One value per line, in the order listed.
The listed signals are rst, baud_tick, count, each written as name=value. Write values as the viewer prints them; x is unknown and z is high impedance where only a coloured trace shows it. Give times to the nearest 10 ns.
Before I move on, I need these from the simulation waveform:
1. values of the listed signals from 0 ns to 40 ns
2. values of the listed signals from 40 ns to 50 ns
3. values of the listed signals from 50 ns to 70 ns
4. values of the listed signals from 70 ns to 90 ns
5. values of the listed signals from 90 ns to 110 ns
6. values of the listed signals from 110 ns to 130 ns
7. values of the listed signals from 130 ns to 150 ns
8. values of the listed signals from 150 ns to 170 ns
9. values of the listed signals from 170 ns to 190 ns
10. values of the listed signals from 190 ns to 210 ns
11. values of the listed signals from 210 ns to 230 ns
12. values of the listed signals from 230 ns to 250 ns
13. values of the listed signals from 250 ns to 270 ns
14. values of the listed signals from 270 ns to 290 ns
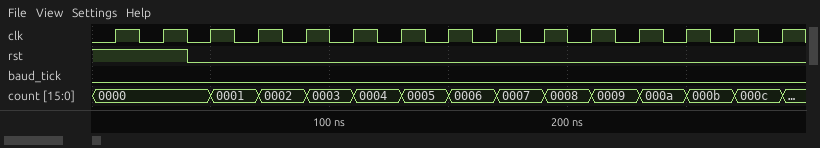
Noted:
rst=1, baud_tick=0, count=0000
rst=0, baud_tick=0, count=0000
rst=0, baud_tick=0, count=0001
rst=0, baud_tick=0, count=0002
rst=0, baud_tick=0, count=0003
rst=0, baud_tick=0, count=0004
rst=0, baud_tick=0, count=0005
rst=0, baud_tick=0, count=0006
rst=0, baud_tick=0, count=0007
rst=0, baud_tick=0, count=0008
rst=0, baud_tick=0, count=0009
rst=0, baud_tick=0, count=000a
rst=0, baud_tick=0, count=000b
rst=0, baud_tick=0, count=000c
